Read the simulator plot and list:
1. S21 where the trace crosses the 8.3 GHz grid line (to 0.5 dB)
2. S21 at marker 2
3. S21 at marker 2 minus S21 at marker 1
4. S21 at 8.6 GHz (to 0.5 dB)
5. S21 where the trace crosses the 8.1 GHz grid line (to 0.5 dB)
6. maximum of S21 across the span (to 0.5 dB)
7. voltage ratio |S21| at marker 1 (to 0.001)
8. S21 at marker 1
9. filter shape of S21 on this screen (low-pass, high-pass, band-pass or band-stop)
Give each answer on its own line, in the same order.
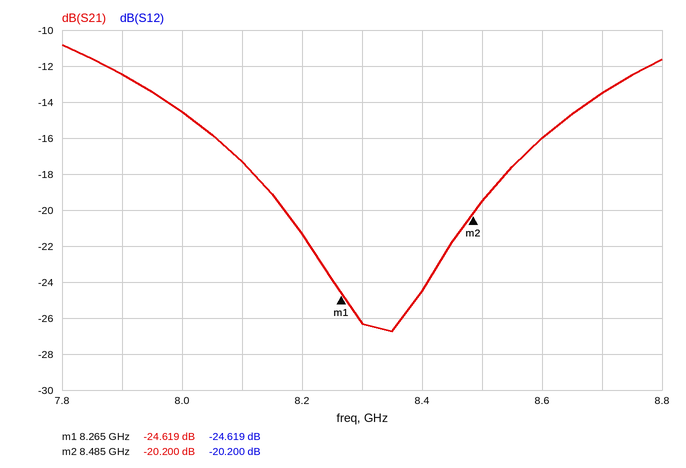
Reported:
-26.5 dB
-20.200 dB
4.419 dB
-16.0 dB
-17.5 dB
-11.0 dB
0.059
-24.619 dB
band-stop
